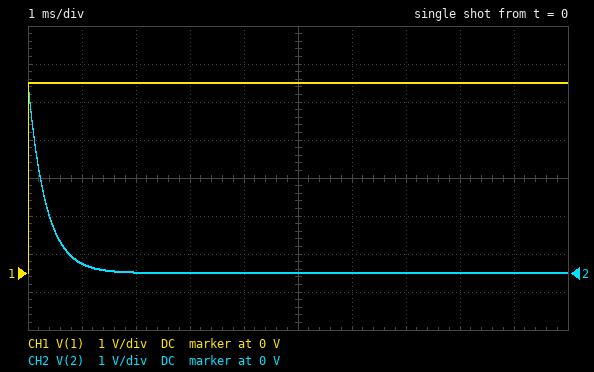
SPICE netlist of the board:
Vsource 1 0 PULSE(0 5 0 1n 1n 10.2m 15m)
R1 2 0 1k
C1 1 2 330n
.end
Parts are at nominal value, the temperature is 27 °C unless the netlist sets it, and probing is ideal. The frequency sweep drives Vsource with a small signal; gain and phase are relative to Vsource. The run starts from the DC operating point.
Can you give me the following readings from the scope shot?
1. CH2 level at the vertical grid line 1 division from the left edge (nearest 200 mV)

200 mV
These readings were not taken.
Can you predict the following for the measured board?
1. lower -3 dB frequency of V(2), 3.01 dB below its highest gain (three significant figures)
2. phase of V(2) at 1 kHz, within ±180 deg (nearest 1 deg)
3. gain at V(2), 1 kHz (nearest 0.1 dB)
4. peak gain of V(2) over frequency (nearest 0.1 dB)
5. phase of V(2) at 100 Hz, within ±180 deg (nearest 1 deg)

482 Hz
26 deg
-0.9 dB
0 dB
78 deg
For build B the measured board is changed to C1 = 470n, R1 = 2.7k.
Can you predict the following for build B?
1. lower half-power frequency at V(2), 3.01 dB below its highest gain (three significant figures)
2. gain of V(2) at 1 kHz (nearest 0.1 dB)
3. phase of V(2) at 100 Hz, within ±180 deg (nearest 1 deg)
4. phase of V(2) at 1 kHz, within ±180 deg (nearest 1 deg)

125 Hz
-0.1 dB
51 deg
7 deg
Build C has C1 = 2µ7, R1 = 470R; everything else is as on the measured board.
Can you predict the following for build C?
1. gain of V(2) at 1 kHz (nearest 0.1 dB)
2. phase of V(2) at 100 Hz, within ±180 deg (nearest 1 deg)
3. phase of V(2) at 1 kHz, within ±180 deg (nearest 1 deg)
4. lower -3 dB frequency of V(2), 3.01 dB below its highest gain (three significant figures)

-0.1 dB
51 deg
7 deg
125 Hz
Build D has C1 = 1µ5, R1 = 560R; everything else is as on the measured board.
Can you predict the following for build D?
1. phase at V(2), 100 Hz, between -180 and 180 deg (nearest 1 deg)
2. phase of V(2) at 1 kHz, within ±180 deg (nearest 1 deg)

62 deg
11 deg
